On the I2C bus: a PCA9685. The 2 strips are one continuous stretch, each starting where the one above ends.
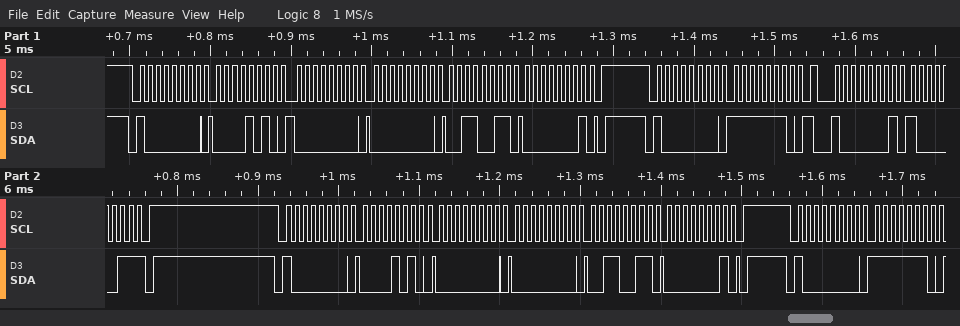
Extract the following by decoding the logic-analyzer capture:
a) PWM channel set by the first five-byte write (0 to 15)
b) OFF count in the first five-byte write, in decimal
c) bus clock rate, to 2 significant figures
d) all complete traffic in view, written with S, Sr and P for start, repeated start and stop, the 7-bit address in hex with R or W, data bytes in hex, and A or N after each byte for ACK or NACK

1
307
100 kHz
S 40W A 0A A 00 A 00 A 33 A 01 A P S 40W A FE A Sr 40R A 83 N P S 40W A 0A A 00 A 00 A 33 A 01 A P S 40W A FE A
